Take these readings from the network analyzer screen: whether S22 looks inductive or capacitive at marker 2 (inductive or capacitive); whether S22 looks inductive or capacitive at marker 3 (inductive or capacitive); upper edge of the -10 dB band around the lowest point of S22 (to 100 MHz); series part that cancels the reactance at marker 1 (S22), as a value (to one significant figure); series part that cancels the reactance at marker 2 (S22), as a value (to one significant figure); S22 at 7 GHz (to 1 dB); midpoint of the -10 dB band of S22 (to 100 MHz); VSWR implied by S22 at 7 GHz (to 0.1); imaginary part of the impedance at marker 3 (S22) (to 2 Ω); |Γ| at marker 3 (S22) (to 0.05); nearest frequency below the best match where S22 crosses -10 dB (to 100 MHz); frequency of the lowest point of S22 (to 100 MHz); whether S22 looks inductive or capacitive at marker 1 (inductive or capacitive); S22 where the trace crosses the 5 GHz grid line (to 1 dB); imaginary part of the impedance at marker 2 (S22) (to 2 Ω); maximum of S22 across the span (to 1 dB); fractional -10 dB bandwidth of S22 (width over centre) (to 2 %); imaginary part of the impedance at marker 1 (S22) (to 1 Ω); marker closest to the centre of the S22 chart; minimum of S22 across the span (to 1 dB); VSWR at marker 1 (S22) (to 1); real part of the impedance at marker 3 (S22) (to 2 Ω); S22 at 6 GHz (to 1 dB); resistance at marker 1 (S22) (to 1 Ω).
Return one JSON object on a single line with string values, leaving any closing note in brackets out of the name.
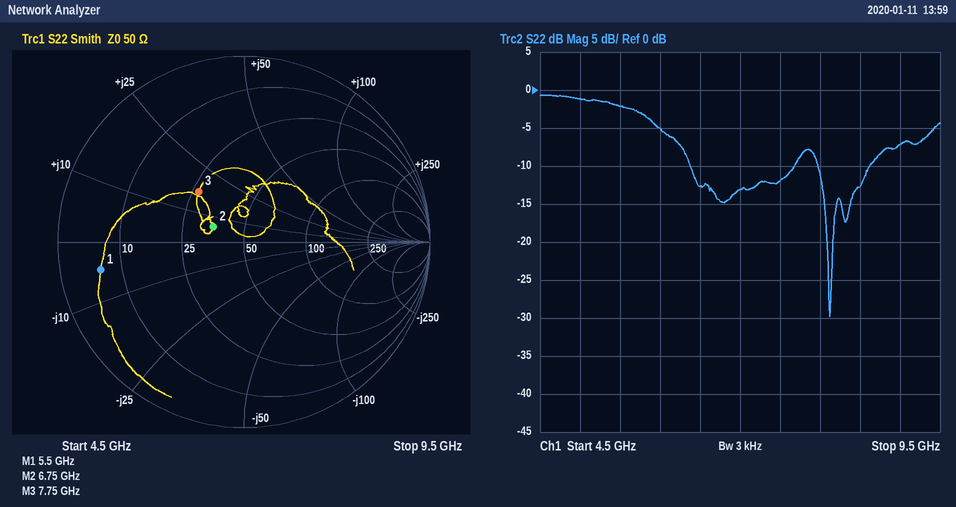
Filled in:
{"whether S22 looks inductive or capacitive at marker 2": "inductive", "whether S22 looks inductive or capacitive at marker 3": "inductive", "upper edge of the -10 dB band around the lowest point of S22": "8.6 GHz", "series part that cancels the reactance at marker 1 (S22), as a value": "100 pH", "series part that cancels the reactance at marker 2 (S22), as a value": "4 pF", "S22 at 7 GHz": "-13 dB", "midpoint of the -10 dB band of S22": "8.3 GHz", "VSWR implied by S22 at 7 GHz": "1.6", "imaginary part of the impedance at marker 3 (S22)": "+16 Ω", "|Γ| at marker 3 (S22)": "0.35", "nearest frequency below the best match where S22 crosses -10 dB": "8.0 GHz", "frequency of the lowest point of S22": "8.1 GHz", "whether S22 looks inductive or capacitive at marker 1": "capacitive", "S22 where the trace crosses the 5 GHz grid line": "-1 dB", "imaginary part of the impedance at marker 2 (S22)": "+6 Ω", "maximum of S22 across the span": "-1 dB", "fractional -10 dB bandwidth of S22 (width over centre)": "8 %", "imaginary part of the impedance at marker 1 (S22)": "-5 Ω", "marker closest to the centre of the S22 chart": "marker 2", "minimum of S22 across the span": "-30 dB", "VSWR at marker 1 (S22)": "8", "real part of the impedance at marker 3 (S22)": "26 Ω", "S22 at 6 GHz": "-5 dB", "resistance at marker 1 (S22)": "6 Ω"}
